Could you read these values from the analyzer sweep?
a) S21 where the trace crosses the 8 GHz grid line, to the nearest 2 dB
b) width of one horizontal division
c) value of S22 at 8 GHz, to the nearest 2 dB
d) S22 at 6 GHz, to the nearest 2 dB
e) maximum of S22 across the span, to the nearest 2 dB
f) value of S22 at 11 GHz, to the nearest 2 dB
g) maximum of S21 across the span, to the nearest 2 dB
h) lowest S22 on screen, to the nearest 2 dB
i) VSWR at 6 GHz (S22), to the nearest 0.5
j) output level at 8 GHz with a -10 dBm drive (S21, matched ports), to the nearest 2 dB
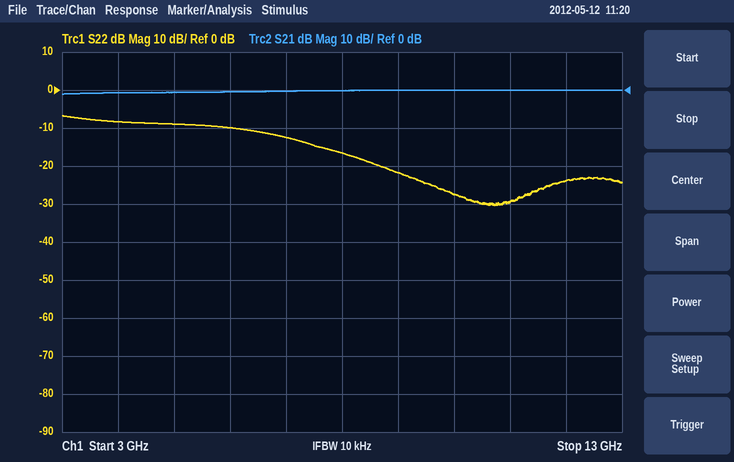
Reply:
0 dB
1 GHz
-16 dB
-10 dB
-6 dB
-30 dB
0 dB
-30 dB
2.0
-10 dBm
